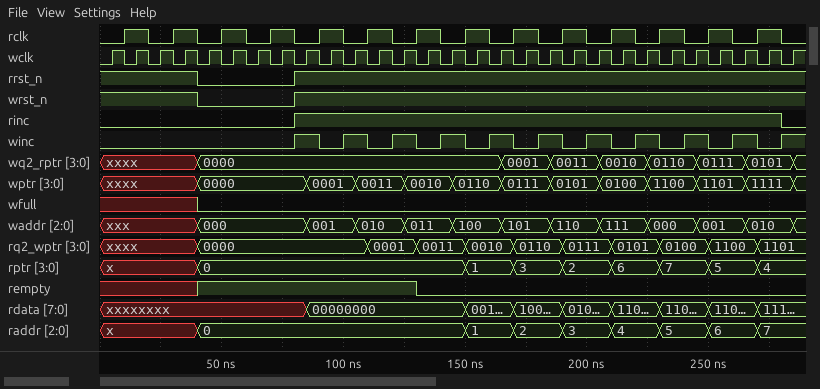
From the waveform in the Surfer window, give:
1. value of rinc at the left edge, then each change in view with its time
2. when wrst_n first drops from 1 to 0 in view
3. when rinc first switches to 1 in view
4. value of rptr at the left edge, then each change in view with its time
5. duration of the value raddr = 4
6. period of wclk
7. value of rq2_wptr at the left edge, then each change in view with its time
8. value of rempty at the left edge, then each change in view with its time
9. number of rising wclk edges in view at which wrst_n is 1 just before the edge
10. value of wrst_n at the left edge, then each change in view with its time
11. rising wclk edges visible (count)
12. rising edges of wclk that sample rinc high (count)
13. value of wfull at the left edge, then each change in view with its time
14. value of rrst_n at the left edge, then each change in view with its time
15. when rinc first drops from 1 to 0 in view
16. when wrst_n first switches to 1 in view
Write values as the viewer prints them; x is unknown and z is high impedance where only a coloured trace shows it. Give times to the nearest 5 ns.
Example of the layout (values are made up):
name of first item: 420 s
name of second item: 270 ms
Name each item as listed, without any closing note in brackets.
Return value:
value of rinc at the left edge, then each change in view with its time: 0, 1 at 80 ns, 0 at 280 ns
when wrst_n first drops from 1 to 0 in view: 40 ns
when rinc first switches to 1 in view: 80 ns
value of rptr at the left edge, then each change in view with its time: x, 0 at 40 ns, 1 at 150 ns, 3 at 170 ns, 2 at 190 ns, 6 at 210 ns, 7 at 230 ns, 5 at 250 ns, 4 at 270 ns
duration of the value raddr = 4: 20 ns
period of wclk: 10 ns
value of rq2_wptr at the left edge, then each change in view with its time: xxxx, 0000 at 40 ns, 0001 at 110 ns, 0011 at 130 ns, 0010 at 150 ns, 0110 at 170 ns, 0111 at 190 ns, 0101 at 210 ns, 0100 at 230 ns, 1100 at 250 ns, 1101 at 270 ns
value of rempty at the left edge, then each change in view with its time: x, 1 at 40 ns, 0 at 130 ns
number of rising wclk edges in view at which wrst_n is 1 just before the edge: 25
value of wrst_n at the left edge, then each change in view with its time: 1, 0 at 40 ns, 1 at 80 ns
rising wclk edges visible: 29
rising edges of wclk that sample rinc high: 20
value of wfull at the left edge, then each change in view with its time: x, 0 at 40 ns
value of rrst_n at the left edge, then each change in view with its time: 1, 0 at 40 ns, 1 at 80 ns
when rinc first drops from 1 to 0 in view: 280 ns
when wrst_n first switches to 1 in view: 80 ns
